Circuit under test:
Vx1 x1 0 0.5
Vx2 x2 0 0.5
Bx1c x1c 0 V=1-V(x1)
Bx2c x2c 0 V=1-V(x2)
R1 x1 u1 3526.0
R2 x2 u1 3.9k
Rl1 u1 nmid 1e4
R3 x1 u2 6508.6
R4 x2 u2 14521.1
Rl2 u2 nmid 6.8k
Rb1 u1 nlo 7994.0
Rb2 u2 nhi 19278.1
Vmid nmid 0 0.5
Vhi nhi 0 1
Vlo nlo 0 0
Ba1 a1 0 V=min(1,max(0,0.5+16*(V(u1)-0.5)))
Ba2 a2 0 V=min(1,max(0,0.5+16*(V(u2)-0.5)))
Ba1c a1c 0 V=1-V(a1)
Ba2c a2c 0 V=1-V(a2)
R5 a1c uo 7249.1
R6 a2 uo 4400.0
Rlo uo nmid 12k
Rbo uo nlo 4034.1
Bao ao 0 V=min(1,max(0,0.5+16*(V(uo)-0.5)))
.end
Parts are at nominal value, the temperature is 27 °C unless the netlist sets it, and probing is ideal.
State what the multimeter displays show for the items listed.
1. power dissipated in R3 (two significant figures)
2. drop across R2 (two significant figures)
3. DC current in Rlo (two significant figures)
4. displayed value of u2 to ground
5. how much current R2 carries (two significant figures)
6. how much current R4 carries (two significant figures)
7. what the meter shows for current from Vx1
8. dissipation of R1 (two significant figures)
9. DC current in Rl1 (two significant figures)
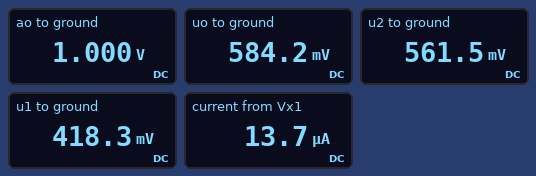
580 nW
82 mV
7.0 µA
561.5 mV
21 µA
4.2 µA
13.7 µA
1.9 µW
8.2 µA
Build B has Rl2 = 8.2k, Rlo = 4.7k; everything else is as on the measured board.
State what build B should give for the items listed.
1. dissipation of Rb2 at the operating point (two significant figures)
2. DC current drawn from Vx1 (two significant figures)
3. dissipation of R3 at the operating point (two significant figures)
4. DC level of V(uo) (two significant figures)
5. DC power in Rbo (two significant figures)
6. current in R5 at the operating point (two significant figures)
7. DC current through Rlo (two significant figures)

9.8 µW
13 µA
660 nW
570 mV
81 µW
59 µA
15 µA
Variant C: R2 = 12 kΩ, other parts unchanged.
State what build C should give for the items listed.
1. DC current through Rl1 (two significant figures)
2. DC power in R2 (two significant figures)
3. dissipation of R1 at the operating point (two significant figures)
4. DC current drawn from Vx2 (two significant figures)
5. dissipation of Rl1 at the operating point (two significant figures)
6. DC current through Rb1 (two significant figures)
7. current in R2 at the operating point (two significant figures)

11 µA
930 nW
3.2 µW
4.6 µA
1.1 µW
49 µA
8.8 µA
